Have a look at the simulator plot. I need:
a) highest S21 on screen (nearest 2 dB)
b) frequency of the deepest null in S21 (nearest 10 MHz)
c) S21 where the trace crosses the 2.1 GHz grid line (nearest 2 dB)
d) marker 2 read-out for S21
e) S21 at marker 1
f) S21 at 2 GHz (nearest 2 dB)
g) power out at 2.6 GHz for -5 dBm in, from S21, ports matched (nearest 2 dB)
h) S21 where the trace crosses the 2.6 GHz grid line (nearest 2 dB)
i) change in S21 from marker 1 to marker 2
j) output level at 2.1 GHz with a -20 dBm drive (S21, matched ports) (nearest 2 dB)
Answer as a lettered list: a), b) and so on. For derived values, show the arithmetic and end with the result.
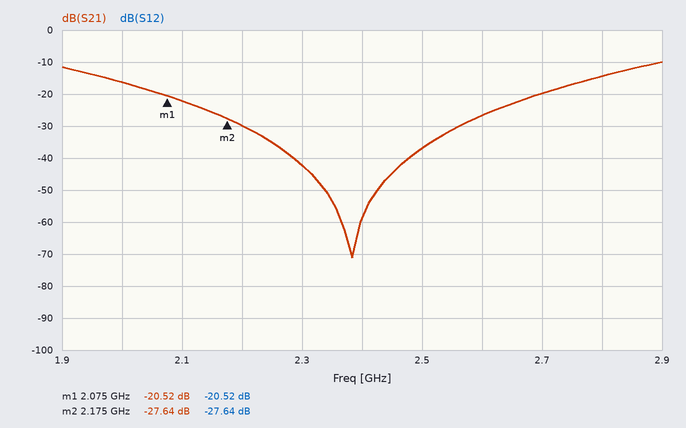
a) -10 dB
b) 2.38 GHz
c) -22 dB
d) -27.64 dB
e) -20.52 dB
f) -16 dB
g) -5 dBm + (-26 dB) = -32 dBm
h) -26 dB
i) -27.64 − (-20.52) = -7.12 dB
j) -20 dBm + (-22 dB) = -42 dBm
